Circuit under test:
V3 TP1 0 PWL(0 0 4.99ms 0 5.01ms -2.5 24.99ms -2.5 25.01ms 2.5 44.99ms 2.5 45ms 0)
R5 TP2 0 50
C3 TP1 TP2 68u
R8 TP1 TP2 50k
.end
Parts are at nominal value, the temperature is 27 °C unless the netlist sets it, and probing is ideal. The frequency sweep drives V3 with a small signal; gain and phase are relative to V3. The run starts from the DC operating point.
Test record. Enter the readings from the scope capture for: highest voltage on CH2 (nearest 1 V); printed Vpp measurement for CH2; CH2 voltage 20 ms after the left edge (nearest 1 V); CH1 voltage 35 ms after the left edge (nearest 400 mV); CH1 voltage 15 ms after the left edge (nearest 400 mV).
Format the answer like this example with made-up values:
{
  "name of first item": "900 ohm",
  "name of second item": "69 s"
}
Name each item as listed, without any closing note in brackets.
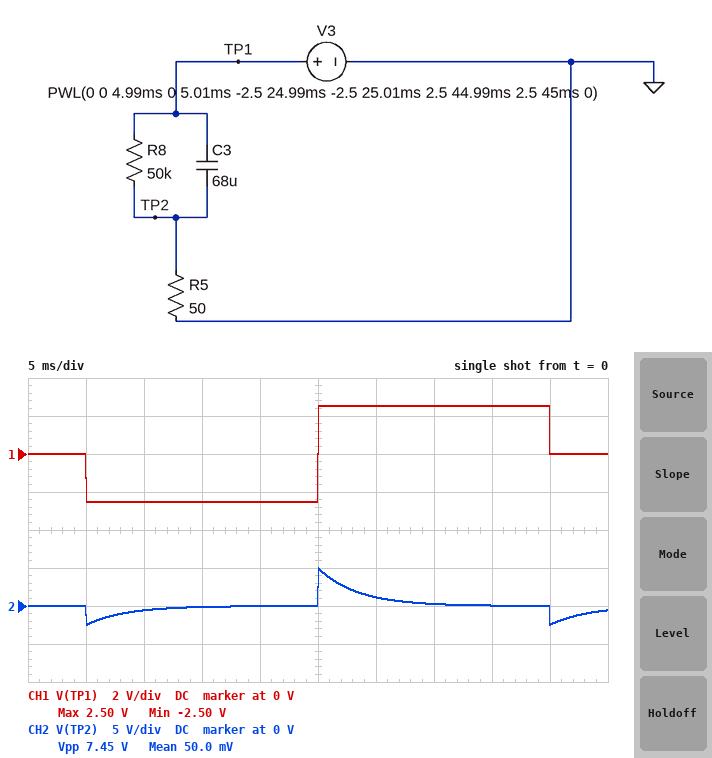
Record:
{
  "highest voltage on CH2": "5 V",
  "printed Vpp measurement for CH2": "7.45 V",
  "CH2 voltage 20 ms after the left edge": "0 V",
  "CH1 voltage 35 ms after the left edge": "2.4 V",
  "CH1 voltage 15 ms after the left edge": "-2.4 V"
}
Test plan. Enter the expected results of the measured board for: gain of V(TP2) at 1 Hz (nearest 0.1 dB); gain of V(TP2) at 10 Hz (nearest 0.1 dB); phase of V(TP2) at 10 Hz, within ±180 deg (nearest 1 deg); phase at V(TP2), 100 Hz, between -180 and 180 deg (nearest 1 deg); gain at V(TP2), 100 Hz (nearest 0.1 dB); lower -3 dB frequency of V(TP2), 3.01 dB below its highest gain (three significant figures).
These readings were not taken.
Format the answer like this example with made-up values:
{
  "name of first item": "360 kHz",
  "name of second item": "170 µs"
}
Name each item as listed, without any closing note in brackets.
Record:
{
  "gain of V(TP2) at 1 Hz": "-33.4 dB",
  "gain of V(TP2) at 10 Hz": "-13.6 dB",
  "phase of V(TP2) at 10 Hz, within ±180 deg": "78 deg",
  "phase at V(TP2), 100 Hz, between -180 and 180 deg": "25 deg",
  "gain at V(TP2), 100 Hz": "-0.9 dB",
  "lower -3 dB frequency of V(TP2), 3.01 dB below its highest gain": "46.9 Hz"
}
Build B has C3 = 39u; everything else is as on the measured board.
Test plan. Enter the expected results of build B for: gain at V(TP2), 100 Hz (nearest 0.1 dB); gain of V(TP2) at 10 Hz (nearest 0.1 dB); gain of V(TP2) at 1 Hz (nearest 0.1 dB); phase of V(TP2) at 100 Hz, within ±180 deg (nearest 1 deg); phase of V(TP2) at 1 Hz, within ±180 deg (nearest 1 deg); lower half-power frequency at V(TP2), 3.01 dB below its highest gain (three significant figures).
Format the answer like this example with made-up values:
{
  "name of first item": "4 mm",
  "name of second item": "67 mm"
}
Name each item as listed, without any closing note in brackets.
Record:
{
  "gain at V(TP2), 100 Hz": "-2.2 dB",
  "gain of V(TP2) at 10 Hz": "-18.3 dB",
  "gain of V(TP2) at 1 Hz": "-38.2 dB",
  "phase of V(TP2) at 100 Hz, within ±180 deg": "39 deg",
  "phase of V(TP2) at 1 Hz, within ±180 deg": "85 deg",
  "lower half-power frequency at V(TP2), 3.01 dB below its highest gain": "81.7 Hz"
}
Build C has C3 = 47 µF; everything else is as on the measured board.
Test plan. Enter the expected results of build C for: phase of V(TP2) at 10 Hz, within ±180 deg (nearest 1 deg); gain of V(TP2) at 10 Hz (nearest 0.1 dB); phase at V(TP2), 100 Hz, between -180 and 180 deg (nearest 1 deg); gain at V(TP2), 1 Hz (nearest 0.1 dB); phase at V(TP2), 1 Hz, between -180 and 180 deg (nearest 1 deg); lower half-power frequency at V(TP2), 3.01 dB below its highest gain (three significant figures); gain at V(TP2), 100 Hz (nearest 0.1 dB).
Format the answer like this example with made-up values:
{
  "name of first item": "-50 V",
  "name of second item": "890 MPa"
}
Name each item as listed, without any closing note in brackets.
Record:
{
  "phase of V(TP2) at 10 Hz, within ±180 deg": "81 deg",
  "gain of V(TP2) at 10 Hz": "-16.7 dB",
  "phase at V(TP2), 100 Hz, between -180 and 180 deg": "34 deg",
  "gain at V(TP2), 1 Hz": "-36.6 dB",
  "phase at V(TP2), 1 Hz, between -180 and 180 deg": "85 deg",
  "lower half-power frequency at V(TP2), 3.01 dB below its highest gain": "67.8 Hz",
  "gain at V(TP2), 100 Hz": "-1.6 dB"
}
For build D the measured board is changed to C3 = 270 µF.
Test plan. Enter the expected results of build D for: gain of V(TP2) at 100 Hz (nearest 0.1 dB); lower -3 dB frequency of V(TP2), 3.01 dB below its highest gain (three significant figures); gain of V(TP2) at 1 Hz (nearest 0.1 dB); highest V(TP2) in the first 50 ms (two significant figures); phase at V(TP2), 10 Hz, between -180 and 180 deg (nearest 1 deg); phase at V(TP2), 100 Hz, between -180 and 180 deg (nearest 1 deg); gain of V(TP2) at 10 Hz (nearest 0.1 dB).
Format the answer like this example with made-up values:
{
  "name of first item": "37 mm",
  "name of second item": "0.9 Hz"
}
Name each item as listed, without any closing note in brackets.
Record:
{
  "gain of V(TP2) at 100 Hz": "-0.1 dB",
  "lower -3 dB frequency of V(TP2), 3.01 dB below its highest gain": "11.8 Hz",
  "gain of V(TP2) at 1 Hz": "-21.5 dB",
  "highest V(TP2) in the first 50 ms": "4.4 V",
  "phase at V(TP2), 10 Hz, between -180 and 180 deg": "50 deg",
  "phase at V(TP2), 100 Hz, between -180 and 180 deg": "7 deg",
  "gain of V(TP2) at 10 Hz": "-3.8 dB"
}
